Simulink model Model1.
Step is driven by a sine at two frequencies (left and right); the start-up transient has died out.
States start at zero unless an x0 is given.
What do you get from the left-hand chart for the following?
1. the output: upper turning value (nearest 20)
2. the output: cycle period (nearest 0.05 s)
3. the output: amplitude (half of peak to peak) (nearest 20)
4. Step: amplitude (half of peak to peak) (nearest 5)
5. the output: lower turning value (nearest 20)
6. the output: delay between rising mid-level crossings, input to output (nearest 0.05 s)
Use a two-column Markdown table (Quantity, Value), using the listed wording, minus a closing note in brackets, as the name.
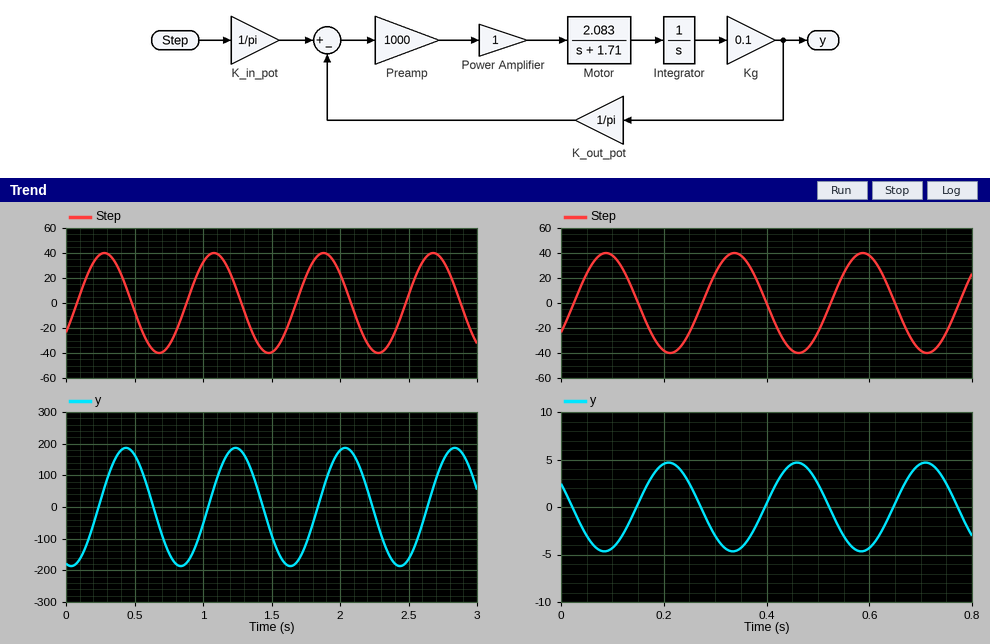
| Quantity | Value |
|---|---|
| the output: upper turning value | 180 |
| the output: cycle period | 0.80 s |
| the output: amplitude (half of peak to peak) | 180 |
| Step: amplitude (half of peak to peak) | 40 |
| the output: lower turning value | -180 |
| the output: delay between rising mid-level crossings, input to output | 0.15 s |
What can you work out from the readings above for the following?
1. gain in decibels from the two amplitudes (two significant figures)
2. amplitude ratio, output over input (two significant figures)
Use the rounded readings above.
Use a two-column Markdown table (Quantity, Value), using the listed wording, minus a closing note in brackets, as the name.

| Quantity | Value |
|---|---|
| gain in decibels from the two amplitudes | 13 dB |
| amplitude ratio, output over input | 4.5 |
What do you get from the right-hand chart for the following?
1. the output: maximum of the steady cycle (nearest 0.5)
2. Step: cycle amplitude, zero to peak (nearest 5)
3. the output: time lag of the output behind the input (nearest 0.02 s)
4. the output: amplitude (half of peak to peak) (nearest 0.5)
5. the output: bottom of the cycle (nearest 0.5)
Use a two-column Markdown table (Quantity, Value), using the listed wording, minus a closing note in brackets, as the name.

| Quantity | Value |
|---|---|
| the output: maximum of the steady cycle | 4.5 |
| Step: cycle amplitude, zero to peak | 40 |
| the output: time lag of the output behind the input | 0.12 s |
| the output: amplitude (half of peak to peak) | 4.5 |
| the output: bottom of the cycle | -4.5 |
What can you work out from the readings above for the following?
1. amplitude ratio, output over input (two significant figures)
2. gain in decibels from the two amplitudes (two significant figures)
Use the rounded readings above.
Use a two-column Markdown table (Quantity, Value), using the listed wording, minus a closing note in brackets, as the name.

| Quantity | Value |
|---|---|
| amplitude ratio, output over input | 0.11 |
| gain in decibels from the two amplitudes | -19 dB |
